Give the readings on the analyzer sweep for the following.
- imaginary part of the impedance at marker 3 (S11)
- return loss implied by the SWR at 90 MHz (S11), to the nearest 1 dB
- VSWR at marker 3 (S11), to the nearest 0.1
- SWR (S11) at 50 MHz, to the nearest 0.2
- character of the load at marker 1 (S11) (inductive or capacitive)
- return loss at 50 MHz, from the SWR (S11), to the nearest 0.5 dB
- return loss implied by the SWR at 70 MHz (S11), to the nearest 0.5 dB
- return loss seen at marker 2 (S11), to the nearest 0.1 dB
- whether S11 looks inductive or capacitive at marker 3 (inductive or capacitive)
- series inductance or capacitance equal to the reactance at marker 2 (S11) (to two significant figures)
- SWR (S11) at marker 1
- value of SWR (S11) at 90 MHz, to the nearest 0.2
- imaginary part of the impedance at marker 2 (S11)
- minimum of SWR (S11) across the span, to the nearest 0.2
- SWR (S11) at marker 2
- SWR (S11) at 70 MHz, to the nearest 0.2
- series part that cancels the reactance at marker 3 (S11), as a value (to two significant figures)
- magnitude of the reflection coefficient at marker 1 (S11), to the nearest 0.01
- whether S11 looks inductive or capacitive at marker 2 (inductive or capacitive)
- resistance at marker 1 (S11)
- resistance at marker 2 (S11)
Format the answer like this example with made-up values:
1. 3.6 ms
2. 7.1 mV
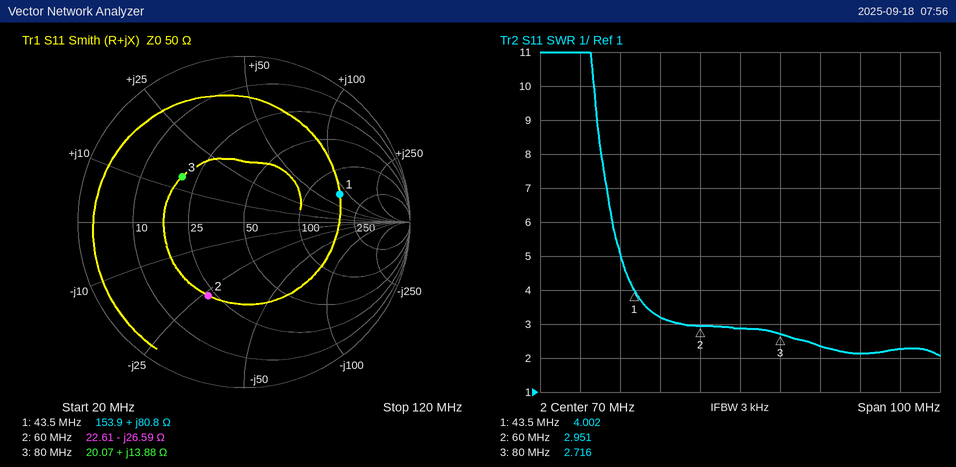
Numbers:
1. +13.88 Ω
2. 8 dB
3. 2.7
4. 3.2
5. inductive
6. 5.5 dB
7. 6.5 dB
8. 6.1 dB
9. inductive
10. 100 pF
11. 4.002
12. 2.4
13. -26.59 Ω
14. 2.0
15. 2.951
16. 2.8
17. 140 pF
18. 0.60
19. capacitive
20. 153.9 Ω
21. 22.61 Ω
